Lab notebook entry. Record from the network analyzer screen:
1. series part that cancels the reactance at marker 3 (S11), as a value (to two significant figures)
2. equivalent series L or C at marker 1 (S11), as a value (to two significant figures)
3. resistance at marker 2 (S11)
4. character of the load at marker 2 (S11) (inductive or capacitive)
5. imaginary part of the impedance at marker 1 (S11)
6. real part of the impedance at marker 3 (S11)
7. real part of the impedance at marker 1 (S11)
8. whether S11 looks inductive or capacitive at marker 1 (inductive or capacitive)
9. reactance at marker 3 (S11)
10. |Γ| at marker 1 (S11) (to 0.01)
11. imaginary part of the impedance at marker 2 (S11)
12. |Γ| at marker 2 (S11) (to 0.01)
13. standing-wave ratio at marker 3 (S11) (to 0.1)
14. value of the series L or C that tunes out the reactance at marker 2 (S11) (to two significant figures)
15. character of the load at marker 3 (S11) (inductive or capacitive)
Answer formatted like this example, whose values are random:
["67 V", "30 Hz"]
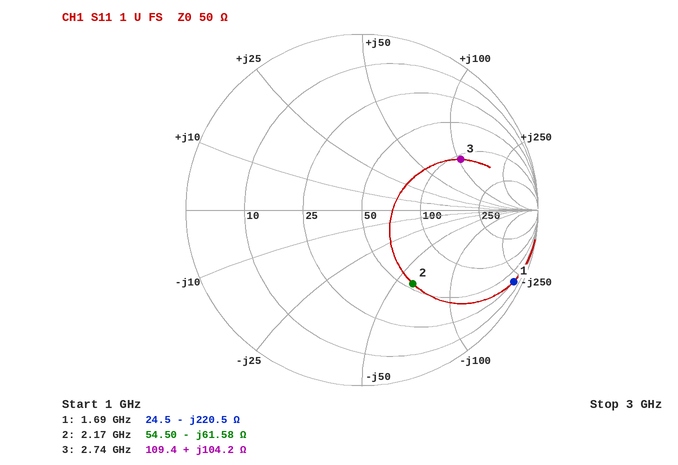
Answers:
["560 fF", "430 fF", "54.50 Ω", "capacitive", "-220.5 Ω", "109.4 Ω", "24.5 Ω", "capacitive", "+104.2 Ω", "0.95", "-61.58 Ω", "0.51", "4.4", "4.5 nH", "inductive"]
